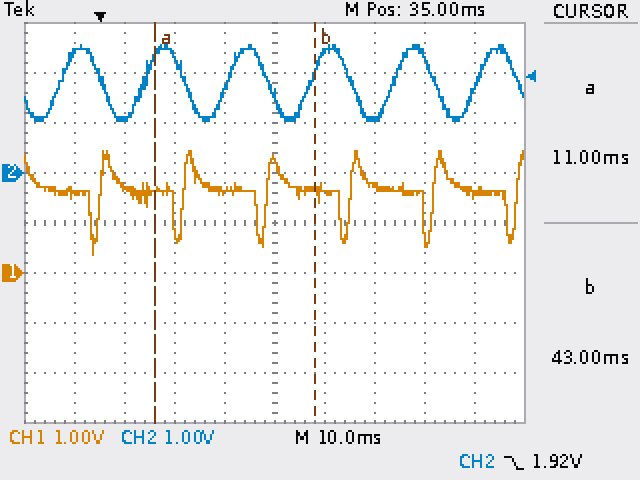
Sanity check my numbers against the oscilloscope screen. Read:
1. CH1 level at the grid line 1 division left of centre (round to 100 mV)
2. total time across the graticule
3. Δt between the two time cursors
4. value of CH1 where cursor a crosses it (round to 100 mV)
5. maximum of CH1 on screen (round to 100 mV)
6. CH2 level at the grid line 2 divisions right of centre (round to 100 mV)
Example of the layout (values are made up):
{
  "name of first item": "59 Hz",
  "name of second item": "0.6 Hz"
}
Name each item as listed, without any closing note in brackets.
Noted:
{
  "CH1 level at the grid line 1 division left of centre": "1.6 V",
  "total time across the graticule": "100 ms",
  "Δt between the two time cursors": "32 ms",
  "value of CH1 where cursor a crosses it": "1.6 V",
  "maximum of CH1 on screen": "2.4 V",
  "CH2 level at the grid line 2 divisions right of centre": "1.1 V"
}
